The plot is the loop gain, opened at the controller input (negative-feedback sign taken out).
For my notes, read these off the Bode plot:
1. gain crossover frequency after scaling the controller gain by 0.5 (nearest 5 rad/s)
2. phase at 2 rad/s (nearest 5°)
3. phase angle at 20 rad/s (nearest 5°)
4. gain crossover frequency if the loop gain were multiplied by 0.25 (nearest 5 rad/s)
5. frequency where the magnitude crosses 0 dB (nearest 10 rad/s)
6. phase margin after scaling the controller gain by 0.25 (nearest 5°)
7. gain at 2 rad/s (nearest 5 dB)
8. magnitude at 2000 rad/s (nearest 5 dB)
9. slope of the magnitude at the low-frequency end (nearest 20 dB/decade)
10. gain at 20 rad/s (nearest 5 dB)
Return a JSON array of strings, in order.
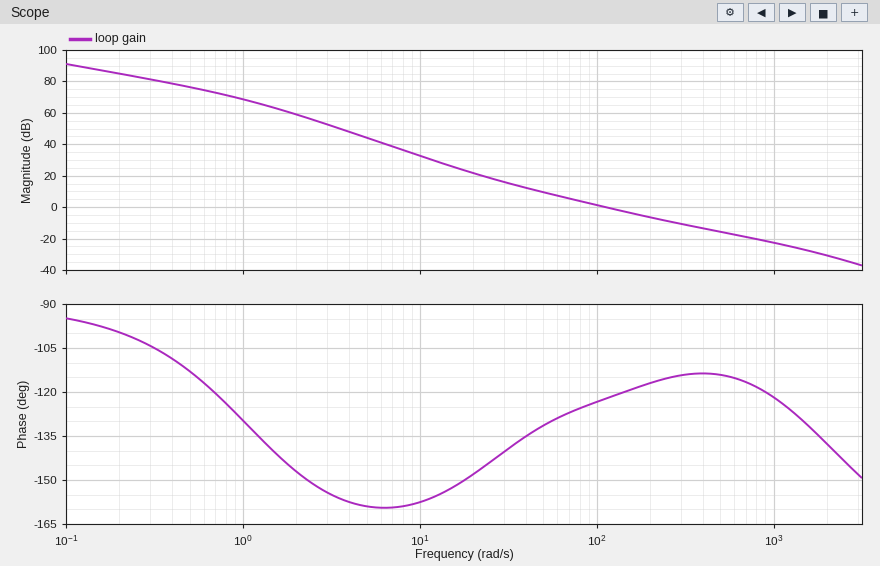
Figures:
["65 rad/s", "-145°", "-150°", "40 rad/s", "110 rad/s", "45°", "60 dB", "-30 dB", "-20 dB/decade", "20 dB"]
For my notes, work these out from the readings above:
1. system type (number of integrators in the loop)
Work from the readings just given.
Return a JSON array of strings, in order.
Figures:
["1"]
